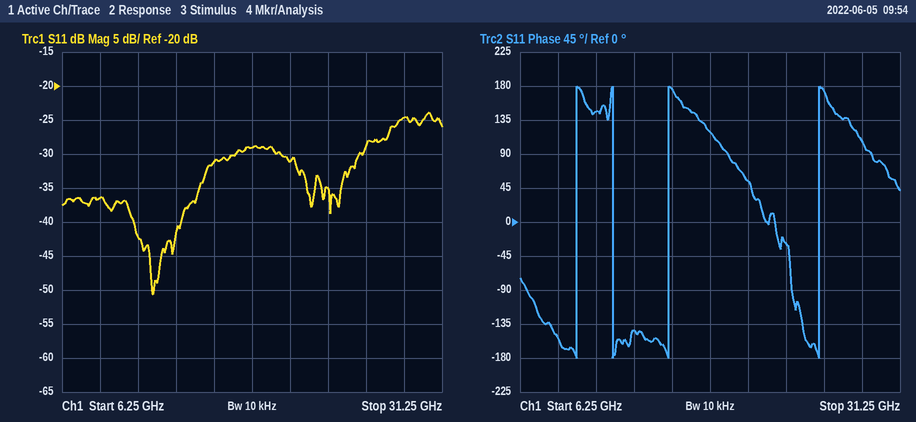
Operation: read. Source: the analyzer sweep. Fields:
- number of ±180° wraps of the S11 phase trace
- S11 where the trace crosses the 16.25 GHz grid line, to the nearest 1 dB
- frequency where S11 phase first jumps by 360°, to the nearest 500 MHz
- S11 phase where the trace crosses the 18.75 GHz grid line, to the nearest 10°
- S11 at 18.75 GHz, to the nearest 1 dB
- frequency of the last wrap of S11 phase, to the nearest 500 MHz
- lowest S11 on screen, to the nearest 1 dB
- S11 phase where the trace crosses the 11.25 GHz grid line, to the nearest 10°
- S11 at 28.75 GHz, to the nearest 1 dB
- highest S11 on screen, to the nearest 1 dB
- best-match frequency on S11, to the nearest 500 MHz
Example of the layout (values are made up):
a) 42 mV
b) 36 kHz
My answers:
a) 4
b) -31 dB
c) 10.0 GHz
d) 120°
e) -29 dB
f) 26.0 GHz
g) -51 dB
h) 150°
i) -25 dB
j) -24 dB
k) 12.0 GHz
